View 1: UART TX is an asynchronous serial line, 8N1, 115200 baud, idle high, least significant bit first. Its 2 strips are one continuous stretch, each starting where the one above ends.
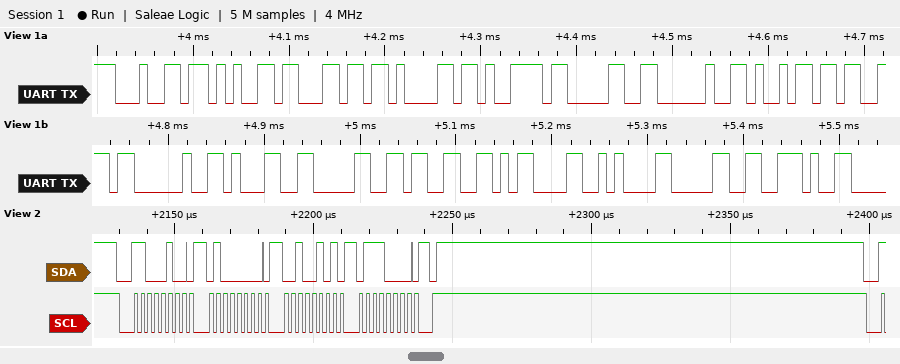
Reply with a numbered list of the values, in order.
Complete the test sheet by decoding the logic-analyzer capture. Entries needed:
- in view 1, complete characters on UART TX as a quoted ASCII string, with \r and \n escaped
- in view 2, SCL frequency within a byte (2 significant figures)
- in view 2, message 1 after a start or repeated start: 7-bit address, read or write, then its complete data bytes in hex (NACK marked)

1. "delay0 is 103\r\n0."
2. 400 kHz
3. 0x62 write: 40 25 70
